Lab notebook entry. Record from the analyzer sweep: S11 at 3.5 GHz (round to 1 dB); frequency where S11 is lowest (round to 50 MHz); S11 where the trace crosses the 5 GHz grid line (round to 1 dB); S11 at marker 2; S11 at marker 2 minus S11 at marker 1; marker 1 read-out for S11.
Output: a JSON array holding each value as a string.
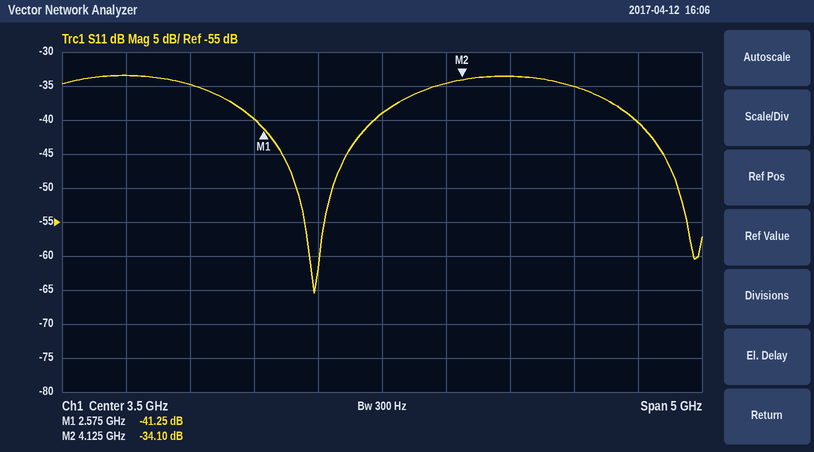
["-39 dB", "2.95 GHz", "-35 dB", "-34.10 dB", "7.15 dB", "-41.25 dB"]
